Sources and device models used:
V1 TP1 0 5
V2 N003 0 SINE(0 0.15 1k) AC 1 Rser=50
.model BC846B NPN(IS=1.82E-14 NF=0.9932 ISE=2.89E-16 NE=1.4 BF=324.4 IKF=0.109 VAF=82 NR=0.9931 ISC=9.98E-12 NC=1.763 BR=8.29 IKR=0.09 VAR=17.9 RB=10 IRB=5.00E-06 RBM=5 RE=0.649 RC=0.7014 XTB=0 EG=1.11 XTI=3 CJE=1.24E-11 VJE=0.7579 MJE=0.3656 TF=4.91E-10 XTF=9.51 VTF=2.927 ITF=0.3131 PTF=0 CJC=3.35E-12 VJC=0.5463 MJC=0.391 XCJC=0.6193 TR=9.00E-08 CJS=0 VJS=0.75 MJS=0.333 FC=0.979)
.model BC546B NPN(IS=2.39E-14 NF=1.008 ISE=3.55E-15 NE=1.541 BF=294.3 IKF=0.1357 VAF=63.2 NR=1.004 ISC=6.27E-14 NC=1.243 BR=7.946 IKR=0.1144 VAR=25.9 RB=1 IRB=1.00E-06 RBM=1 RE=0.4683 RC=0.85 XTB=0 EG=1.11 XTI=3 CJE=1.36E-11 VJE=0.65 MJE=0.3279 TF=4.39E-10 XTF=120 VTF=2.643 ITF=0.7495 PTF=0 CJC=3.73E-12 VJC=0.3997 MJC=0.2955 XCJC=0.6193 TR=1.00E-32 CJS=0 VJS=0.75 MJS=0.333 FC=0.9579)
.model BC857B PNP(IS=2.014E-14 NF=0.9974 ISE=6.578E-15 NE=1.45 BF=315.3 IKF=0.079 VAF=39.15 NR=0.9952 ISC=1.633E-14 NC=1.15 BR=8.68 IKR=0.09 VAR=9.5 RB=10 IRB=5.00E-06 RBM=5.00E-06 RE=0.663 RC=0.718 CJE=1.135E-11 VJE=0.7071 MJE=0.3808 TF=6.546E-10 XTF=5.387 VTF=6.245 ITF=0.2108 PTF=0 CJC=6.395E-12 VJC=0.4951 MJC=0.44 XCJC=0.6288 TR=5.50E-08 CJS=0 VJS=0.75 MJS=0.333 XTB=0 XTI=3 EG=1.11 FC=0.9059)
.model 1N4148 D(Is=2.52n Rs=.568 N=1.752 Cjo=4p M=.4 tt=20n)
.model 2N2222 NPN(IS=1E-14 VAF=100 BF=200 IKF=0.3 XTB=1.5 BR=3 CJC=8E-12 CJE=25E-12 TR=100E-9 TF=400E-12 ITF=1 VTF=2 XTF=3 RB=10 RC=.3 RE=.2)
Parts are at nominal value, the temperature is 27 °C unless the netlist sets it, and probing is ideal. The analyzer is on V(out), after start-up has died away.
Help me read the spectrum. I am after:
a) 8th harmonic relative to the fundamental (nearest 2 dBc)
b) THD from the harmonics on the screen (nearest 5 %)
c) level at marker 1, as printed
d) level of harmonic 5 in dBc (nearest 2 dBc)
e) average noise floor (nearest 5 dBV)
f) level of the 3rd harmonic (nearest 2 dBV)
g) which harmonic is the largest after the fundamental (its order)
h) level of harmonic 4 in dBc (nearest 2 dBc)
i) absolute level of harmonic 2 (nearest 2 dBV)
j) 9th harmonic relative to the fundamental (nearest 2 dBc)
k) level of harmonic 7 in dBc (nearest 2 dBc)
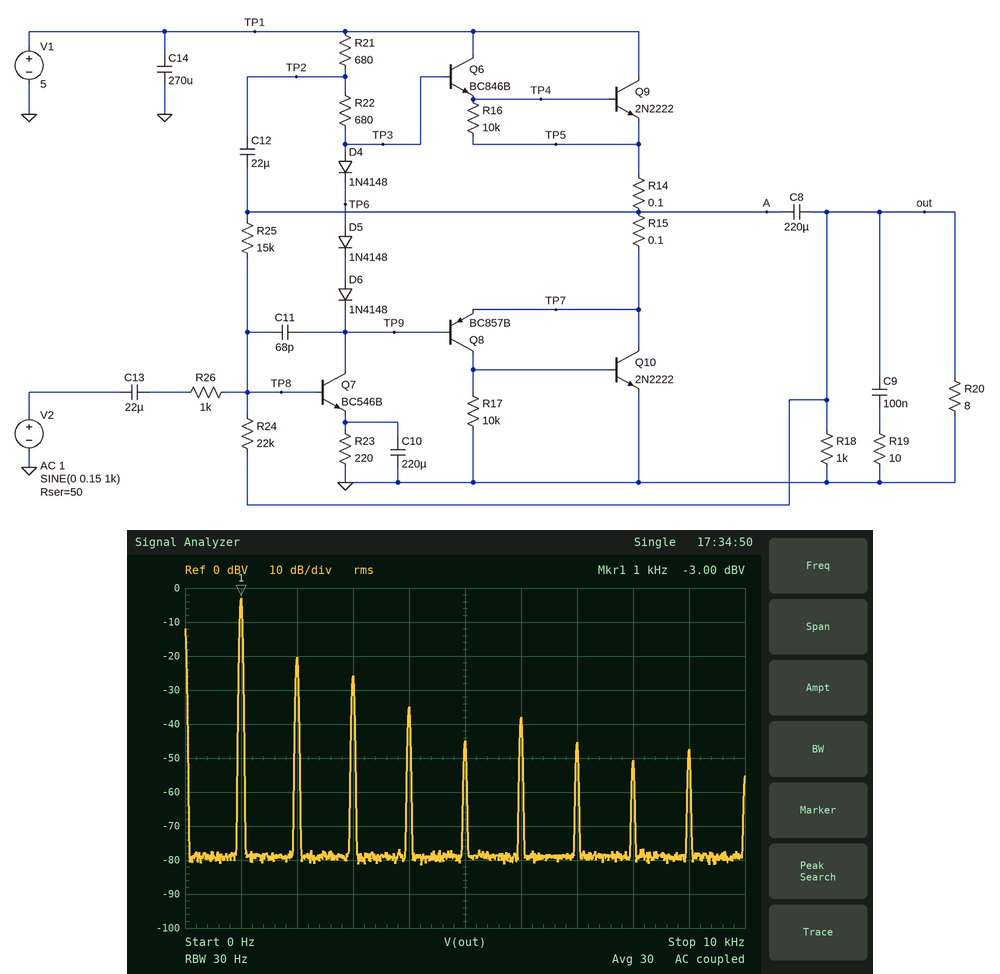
-48 dBc
15 %
-3.00 dBV
-42 dBc
-80 dBV
-26 dBV
2
-32 dBc
-20 dBV
-44 dBc
-42 dBc
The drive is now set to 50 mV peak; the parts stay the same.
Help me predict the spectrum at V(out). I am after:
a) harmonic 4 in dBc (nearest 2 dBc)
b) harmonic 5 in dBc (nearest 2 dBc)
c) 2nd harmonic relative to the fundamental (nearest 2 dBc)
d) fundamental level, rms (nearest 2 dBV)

-46 dBc
-50 dBc
-38 dBc
-12 dBV
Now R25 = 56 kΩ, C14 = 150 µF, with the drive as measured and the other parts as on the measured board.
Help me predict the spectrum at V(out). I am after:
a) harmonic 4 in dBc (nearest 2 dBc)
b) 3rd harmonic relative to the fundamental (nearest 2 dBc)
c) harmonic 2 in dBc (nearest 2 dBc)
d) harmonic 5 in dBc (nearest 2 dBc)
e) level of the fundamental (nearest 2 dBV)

-34 dBc
-26 dBc
-18 dBc
-32 dBc
2 dBV
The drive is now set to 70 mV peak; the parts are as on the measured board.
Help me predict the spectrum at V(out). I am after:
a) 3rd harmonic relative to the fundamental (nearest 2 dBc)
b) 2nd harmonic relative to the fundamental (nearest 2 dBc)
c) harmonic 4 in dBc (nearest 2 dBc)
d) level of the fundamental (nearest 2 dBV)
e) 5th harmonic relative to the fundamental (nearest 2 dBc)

-42 dBc
-40 dBc
-48 dBc
-8 dBV
-48 dBc
